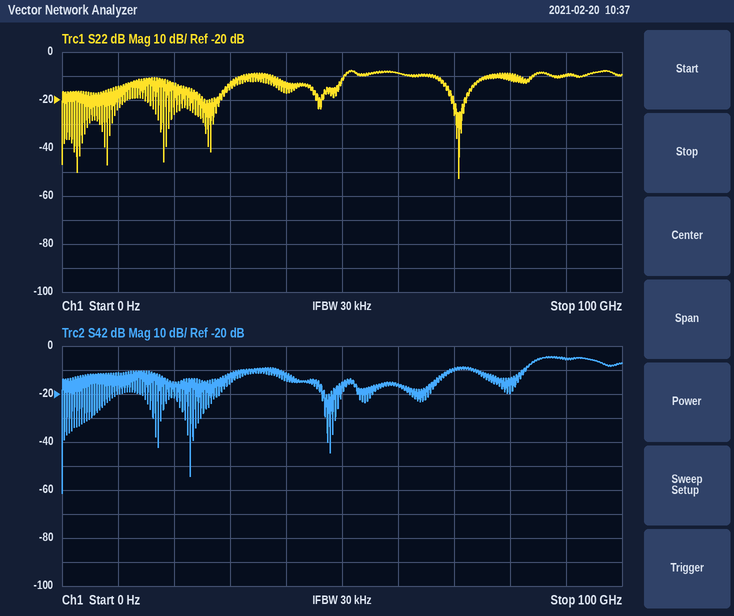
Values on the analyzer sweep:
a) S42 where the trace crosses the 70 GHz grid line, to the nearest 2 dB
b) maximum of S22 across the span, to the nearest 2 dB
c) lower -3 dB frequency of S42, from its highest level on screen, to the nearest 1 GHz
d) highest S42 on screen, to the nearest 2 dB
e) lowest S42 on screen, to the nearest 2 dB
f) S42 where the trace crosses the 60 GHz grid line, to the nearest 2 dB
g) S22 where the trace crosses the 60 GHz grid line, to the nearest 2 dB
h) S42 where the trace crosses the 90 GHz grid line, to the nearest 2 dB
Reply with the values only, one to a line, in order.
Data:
-10 dB
-8 dB
84 GHz
-4 dB
-62 dB
-16 dB
-8 dB
-6 dB
